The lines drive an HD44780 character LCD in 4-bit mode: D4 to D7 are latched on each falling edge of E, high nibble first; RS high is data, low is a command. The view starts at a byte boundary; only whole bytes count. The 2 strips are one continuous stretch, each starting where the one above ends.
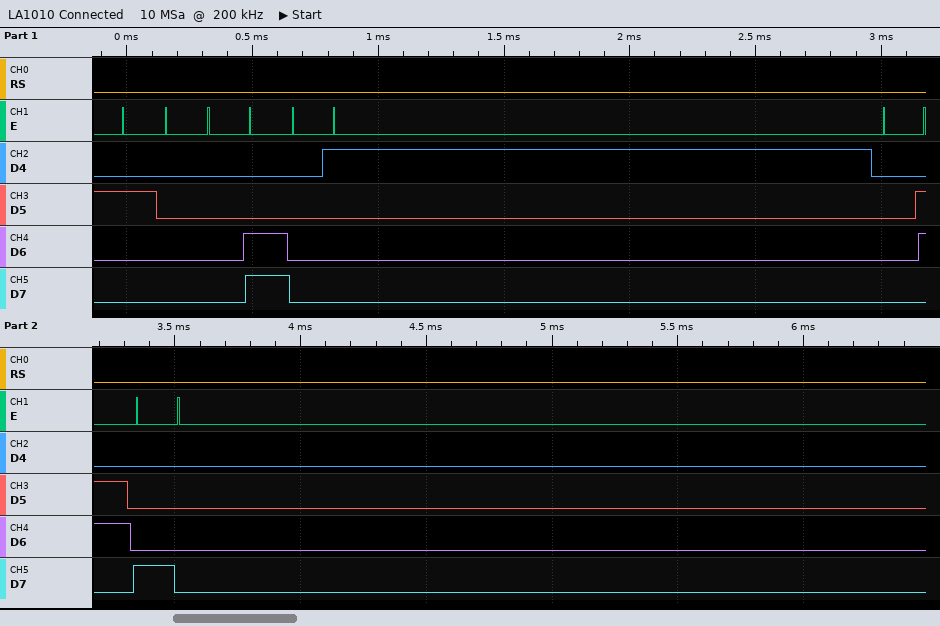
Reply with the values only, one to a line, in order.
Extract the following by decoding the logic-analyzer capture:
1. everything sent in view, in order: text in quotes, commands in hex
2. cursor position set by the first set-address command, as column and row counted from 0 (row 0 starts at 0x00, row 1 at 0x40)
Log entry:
0x20 0x0C 0x01 0x06 0x80
column 0, row 0
